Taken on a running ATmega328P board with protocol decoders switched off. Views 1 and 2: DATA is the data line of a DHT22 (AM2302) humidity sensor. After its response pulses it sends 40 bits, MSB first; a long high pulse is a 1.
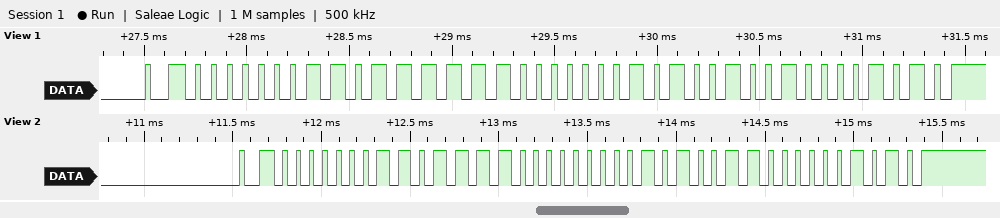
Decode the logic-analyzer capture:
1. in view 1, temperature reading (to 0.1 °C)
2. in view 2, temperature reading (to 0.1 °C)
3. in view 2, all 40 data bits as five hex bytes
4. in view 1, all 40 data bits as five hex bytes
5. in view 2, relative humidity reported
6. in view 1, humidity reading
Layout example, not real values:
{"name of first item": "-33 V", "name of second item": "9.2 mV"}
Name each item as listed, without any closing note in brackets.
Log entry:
{"in view 1, temperature reading": "32.9 °C", "in view 2, temperature reading": "33.2 °C", "in view 2, all 40 data bits as five hex bytes": "01 BC 01 4C 0A", "in view 1, all 40 data bits as five hex bytes": "01 BF 01 49 0A", "in view 2, relative humidity reported": "44.4 %", "in view 1, humidity reading": "44.7 %"}
